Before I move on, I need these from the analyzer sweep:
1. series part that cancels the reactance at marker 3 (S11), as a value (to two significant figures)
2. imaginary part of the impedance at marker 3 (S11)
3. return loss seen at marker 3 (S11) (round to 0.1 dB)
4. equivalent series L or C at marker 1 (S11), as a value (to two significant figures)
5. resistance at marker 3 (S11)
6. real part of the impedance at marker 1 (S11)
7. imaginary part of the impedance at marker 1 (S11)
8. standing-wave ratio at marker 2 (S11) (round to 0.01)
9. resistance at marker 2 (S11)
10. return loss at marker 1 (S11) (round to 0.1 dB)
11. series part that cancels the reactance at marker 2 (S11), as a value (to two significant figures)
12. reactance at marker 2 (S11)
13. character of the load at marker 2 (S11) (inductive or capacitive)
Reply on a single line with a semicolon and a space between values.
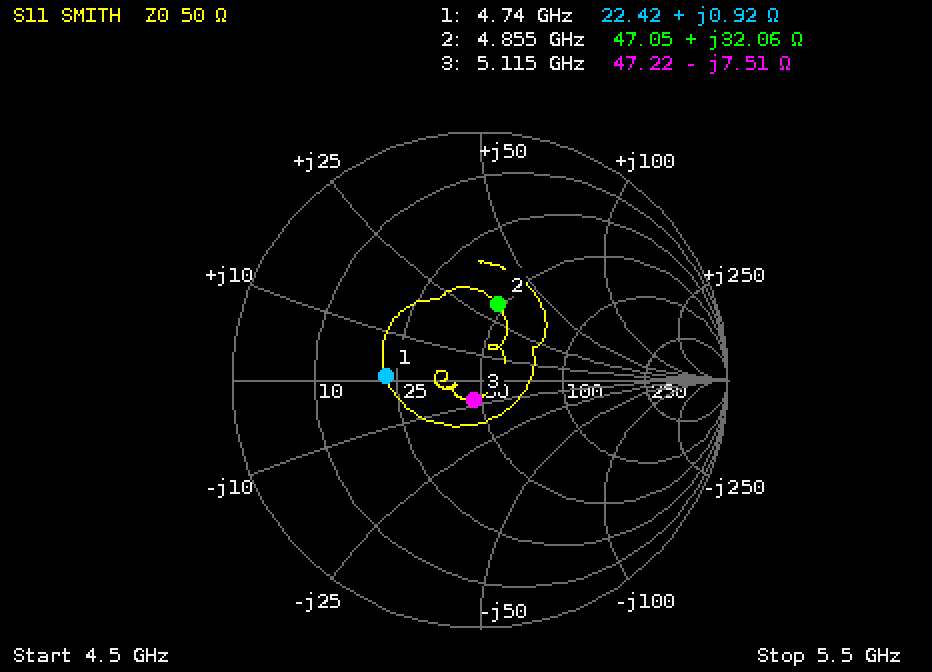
230 pH; -7.51 Ω; 21.7 dB; 31 pH; 47.22 Ω; 22.42 Ω; +0.92 Ω; 1.92; 47.05 Ω; 8.4 dB; 1.0 pF; +32.06 Ω; inductive
